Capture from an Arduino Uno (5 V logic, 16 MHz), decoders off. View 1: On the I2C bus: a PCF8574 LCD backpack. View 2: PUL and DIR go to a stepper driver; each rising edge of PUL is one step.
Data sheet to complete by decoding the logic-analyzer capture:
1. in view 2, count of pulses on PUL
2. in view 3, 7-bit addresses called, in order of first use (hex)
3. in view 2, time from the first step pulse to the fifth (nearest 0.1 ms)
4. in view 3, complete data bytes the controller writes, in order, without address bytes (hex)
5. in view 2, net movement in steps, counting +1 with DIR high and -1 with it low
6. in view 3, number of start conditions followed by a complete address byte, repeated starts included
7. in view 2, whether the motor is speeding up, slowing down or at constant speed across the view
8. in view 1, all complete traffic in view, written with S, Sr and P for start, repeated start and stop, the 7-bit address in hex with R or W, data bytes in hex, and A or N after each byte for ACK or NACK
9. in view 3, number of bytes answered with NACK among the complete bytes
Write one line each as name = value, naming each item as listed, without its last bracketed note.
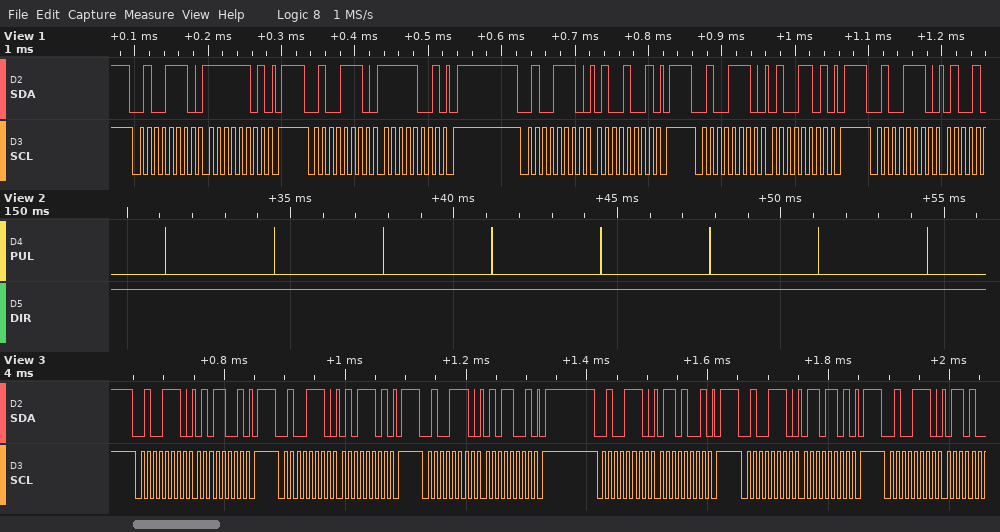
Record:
in view 2, count of pulses on PUL = 8
in view 3, 7-bit addresses called, in order of first use = 0x27
in view 2, time from the first step pulse to the fifth = 13.3 ms
in view 3, complete data bytes the controller writes, in order, without address bytes = 59 5D 59 69 6D
in view 2, net movement in steps, counting +1 with DIR high and -1 with it low = +8
in view 3, number of start conditions followed by a complete address byte, repeated starts included = 6
in view 2, whether the motor is speeding up, slowing down or at constant speed across the view = constant speed
in view 1, all complete traffic in view, written with S, Sr and P for start, repeated start and stop, the 7-bit address in hex with R or W, data bytes in hex, and A or N after each byte for ACK or NACK = S 27W A FD A P S 27W A F9 A P S 27W A 49 A P S 27W A 4D A P S 27W A
in view 3, number of bytes answered with NACK among the complete bytes = 0
